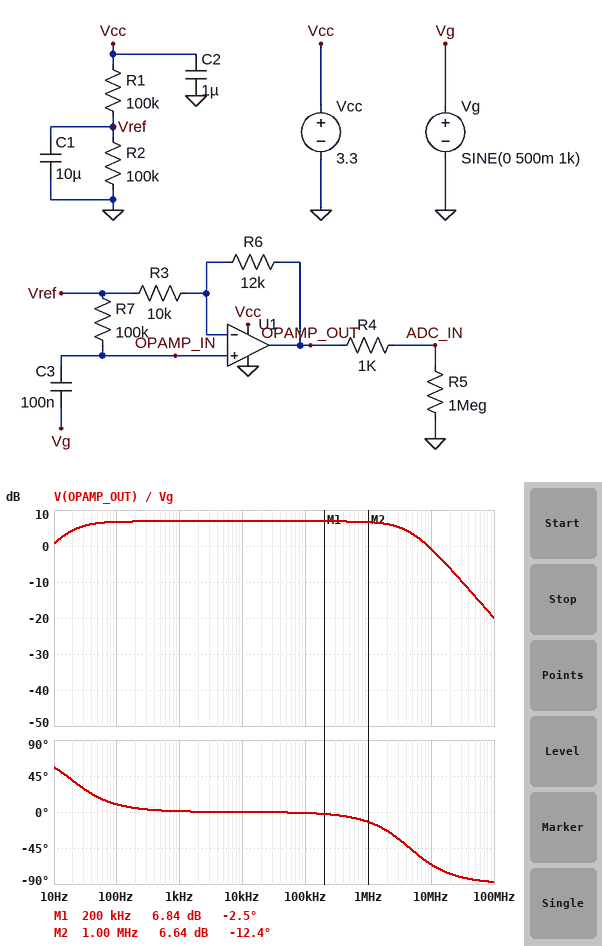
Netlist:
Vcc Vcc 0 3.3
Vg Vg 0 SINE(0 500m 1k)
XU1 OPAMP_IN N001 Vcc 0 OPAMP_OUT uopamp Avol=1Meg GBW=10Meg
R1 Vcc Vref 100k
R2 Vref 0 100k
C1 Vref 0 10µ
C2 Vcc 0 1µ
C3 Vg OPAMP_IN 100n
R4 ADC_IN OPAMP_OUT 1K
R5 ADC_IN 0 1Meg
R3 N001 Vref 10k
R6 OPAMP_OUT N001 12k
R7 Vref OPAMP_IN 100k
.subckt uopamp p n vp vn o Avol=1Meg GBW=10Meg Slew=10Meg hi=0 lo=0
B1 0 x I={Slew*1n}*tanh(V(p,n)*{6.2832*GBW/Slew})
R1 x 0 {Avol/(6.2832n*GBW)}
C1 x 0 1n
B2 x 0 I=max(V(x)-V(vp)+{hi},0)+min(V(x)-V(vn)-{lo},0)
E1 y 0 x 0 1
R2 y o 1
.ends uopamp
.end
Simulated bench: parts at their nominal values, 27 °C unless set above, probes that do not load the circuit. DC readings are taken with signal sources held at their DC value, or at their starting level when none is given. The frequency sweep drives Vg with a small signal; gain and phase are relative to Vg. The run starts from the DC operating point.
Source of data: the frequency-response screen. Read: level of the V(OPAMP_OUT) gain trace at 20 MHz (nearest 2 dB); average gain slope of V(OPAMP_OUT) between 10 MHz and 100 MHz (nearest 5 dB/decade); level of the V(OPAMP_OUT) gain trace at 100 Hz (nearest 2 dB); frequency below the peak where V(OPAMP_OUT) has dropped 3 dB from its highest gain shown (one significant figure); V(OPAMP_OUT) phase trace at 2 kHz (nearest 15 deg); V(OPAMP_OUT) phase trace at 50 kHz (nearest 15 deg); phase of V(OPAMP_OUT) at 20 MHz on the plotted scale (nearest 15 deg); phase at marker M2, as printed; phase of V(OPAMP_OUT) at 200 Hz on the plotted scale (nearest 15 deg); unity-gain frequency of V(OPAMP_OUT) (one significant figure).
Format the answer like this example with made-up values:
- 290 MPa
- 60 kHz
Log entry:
- -6 dB
- -20 dB/decade
- 6 dB
- 20 Hz
- 0 deg
- 0 deg
- -75 deg
- -12.4 deg
- 0 deg
- 9 MHz
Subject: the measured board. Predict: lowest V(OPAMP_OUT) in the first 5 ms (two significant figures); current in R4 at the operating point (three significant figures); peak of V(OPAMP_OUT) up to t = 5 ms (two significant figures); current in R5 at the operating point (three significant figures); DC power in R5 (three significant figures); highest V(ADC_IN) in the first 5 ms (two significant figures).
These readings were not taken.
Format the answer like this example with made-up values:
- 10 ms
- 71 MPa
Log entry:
- 530 mV
- 1.65 µA
- 2.7 V
- 1.65 µA
- 2.72 µW
- 2.7 V
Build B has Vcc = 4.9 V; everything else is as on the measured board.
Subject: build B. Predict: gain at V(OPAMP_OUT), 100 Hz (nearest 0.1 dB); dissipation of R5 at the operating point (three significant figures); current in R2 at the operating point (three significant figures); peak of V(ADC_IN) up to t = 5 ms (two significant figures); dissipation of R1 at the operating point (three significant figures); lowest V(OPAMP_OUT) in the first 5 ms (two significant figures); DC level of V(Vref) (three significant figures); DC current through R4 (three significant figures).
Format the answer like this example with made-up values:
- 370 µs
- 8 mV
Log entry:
- 6.7 dB
- 5.99 µW
- 24.5 µA
- 3.5 V
- 60.0 µW
- 1.3 V
- 2.45 V
- 2.45 µA
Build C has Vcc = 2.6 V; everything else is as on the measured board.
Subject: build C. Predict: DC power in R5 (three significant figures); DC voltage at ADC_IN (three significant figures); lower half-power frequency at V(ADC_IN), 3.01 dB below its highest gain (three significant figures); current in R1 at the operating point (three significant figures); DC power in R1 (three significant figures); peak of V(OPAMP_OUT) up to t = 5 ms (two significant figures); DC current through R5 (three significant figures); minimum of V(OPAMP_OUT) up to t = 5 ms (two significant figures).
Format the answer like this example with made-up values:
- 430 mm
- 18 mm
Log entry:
- 1.69 µW
- 1.30 V
- 17.6 Hz
- 13.0 µA
- 16.9 µW
- 2.4 V
- 1.30 µA
- 180 mV
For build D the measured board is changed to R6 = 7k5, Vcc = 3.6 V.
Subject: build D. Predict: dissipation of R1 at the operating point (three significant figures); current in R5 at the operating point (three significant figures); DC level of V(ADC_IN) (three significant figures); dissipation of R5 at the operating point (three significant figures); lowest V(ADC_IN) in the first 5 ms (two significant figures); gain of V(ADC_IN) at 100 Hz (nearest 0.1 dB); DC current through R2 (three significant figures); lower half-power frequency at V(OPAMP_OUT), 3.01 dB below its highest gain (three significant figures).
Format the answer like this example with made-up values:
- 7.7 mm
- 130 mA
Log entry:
- 32.4 µW
- 1.80 µA
- 1.80 V
- 3.23 µW
- 910 mV
- 4.7 dB
- 18.0 µA
- 17.6 Hz
